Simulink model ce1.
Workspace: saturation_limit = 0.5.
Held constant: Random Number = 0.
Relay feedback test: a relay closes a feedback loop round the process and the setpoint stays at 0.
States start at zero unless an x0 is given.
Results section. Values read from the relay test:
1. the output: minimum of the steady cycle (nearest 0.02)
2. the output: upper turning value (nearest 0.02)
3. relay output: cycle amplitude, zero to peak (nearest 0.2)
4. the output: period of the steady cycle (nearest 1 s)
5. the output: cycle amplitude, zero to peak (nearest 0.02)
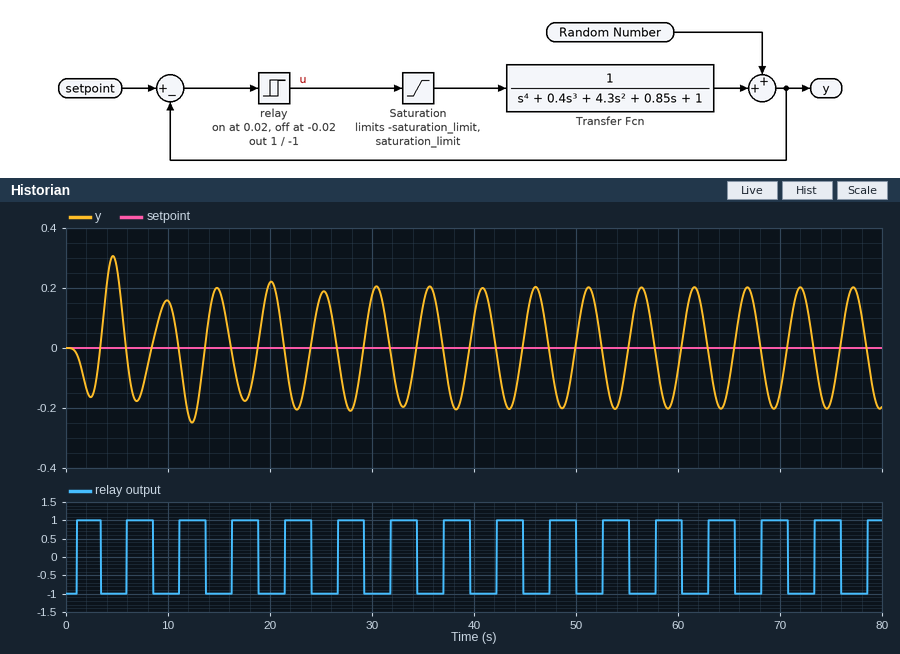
-0.20
0.20
1.0
5 s
0.20
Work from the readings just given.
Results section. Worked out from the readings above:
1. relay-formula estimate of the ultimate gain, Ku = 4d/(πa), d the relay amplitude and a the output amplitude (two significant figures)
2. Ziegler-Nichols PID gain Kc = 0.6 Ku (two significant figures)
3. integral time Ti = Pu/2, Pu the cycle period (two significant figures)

6.4
3.8
2.5 s
